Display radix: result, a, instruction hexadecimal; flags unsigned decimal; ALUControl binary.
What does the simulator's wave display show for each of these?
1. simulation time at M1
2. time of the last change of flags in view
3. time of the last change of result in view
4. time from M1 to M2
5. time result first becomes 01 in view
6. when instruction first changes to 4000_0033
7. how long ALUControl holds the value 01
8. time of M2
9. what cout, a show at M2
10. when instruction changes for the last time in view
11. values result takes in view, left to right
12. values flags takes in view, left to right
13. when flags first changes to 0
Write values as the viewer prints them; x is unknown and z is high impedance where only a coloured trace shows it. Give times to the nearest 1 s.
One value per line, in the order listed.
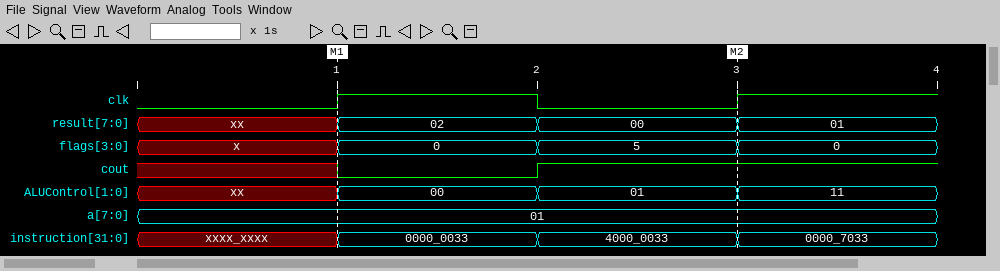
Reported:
1 s
3 s
3 s
2 s
3 s
2 s
1 s
3 s
cout=1, a=01
3 s
xx, 02, 00, 01
x, 0, 5, 0
1 s
